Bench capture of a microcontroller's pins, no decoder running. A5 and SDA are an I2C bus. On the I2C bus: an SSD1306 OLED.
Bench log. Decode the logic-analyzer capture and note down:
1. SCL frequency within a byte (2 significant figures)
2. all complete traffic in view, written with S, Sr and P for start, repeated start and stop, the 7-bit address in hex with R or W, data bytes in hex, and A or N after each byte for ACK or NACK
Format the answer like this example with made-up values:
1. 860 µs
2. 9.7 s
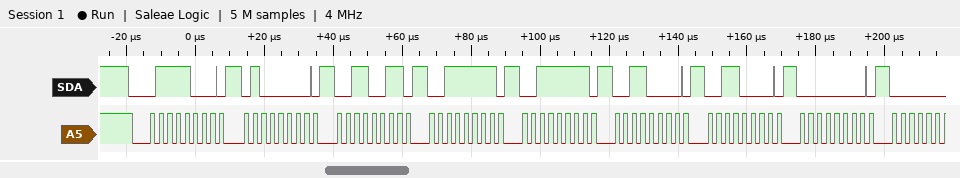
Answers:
1. 400 kHz
2. S 3CW A 40 A 33 A 3F A 3F A 30 A 30 A 00 A
